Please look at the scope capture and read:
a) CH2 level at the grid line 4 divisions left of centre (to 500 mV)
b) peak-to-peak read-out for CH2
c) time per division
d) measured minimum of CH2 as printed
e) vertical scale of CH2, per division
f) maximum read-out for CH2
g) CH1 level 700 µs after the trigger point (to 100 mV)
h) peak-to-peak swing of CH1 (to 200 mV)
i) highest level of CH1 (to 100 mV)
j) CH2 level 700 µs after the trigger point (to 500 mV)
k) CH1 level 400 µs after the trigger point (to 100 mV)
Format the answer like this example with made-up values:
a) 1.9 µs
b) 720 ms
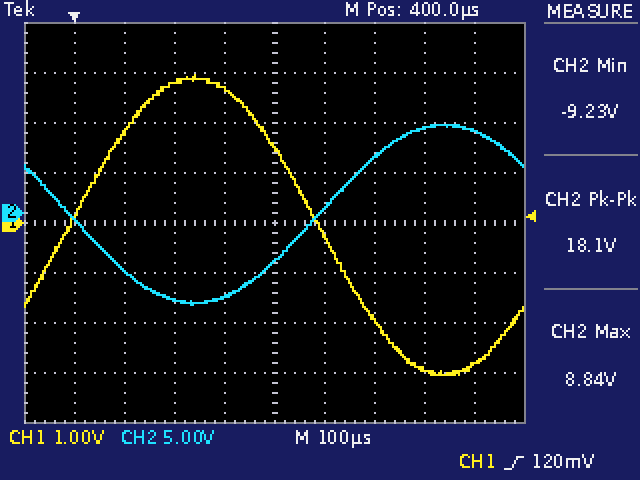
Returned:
a) -500 mV
b) 18.1 V
c) 100 µs
d) -9.23 V
e) 5 V
f) 8.84 V
g) -2.9 V
h) 6.0 V
i) 3.0 V
j) 8.5 V
k) 1.5 V
